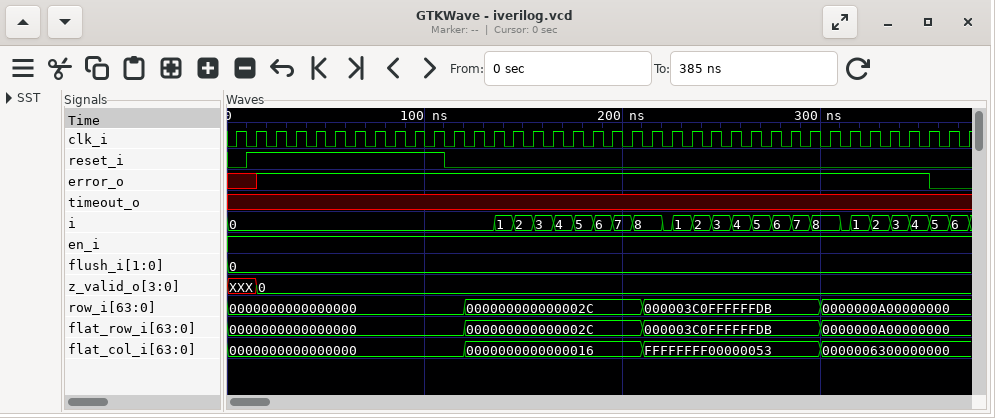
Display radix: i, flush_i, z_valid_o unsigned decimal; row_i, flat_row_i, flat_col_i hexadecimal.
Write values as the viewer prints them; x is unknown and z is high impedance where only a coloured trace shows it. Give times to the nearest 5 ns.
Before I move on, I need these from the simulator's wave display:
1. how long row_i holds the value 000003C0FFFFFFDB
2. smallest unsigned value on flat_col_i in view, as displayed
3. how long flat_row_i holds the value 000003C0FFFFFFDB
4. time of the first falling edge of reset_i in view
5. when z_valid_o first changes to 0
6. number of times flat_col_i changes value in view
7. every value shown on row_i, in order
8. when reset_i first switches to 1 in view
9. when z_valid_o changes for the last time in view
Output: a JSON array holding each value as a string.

["90 ns", "0000000000000000", "90 ns", "110 ns", "15 ns", "3", "0000000000000000, 000000000000002C, 000003C0FFFFFFDB, 0000000A00000000", "10 ns", "15 ns"]
